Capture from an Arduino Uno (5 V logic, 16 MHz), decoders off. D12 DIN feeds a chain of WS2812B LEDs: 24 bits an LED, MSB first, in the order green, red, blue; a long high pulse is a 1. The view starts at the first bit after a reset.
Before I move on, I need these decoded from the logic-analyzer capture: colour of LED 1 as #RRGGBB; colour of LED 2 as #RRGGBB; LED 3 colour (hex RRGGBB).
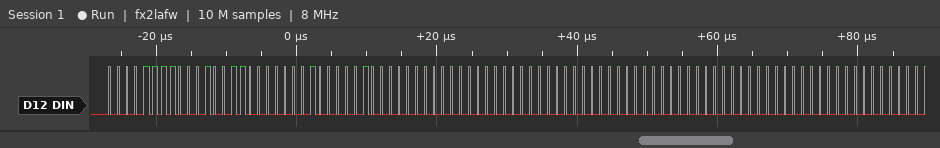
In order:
#130F01
#000400
#000000
